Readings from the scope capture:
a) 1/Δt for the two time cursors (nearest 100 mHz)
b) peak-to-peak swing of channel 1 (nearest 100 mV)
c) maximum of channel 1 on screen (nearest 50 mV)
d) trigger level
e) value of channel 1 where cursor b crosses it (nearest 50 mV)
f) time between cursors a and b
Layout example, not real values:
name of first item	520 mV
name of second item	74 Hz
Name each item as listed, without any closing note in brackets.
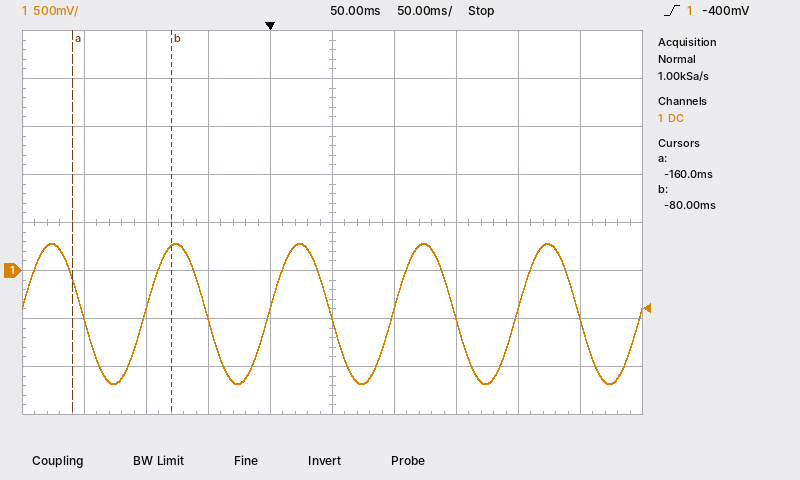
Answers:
1/Δt for the two time cursors	12.5 Hz
peak-to-peak swing of channel 1	1.50 V
maximum of channel 1 on screen	300 mV
trigger level	-400 mV
value of channel 1 where cursor b crosses it	250 mV
time between cursors a and b	80 ms
